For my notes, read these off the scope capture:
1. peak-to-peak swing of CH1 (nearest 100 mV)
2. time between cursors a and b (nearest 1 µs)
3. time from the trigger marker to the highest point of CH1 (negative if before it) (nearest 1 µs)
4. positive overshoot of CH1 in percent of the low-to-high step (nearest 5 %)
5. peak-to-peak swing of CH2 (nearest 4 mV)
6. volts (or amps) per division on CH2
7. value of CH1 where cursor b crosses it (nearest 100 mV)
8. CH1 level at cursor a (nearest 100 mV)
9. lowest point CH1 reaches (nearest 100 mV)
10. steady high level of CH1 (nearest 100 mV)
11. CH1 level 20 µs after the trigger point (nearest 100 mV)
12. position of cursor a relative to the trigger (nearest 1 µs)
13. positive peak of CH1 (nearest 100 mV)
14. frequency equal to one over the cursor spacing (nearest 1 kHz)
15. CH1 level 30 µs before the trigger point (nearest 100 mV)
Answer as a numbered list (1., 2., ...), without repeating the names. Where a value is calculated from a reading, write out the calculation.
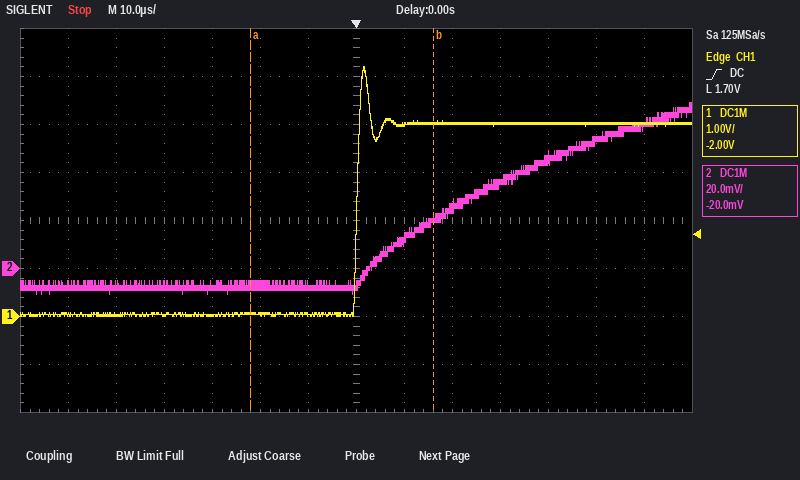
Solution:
1. 5.2 V − (0.0 V) = 5.2 V
2. 38 µs
3. +2 µs
4. 30 %
5. 80 mV
6. 20 mV
7. 4.0 V
8. 100 mV
9. 0.0 V
10. 4.0 V
11. 4.0 V
12. -22 µs
13. 5.2 V
14. 1 / 38 µs ≈ 26 kHz
15. 0.0 V
